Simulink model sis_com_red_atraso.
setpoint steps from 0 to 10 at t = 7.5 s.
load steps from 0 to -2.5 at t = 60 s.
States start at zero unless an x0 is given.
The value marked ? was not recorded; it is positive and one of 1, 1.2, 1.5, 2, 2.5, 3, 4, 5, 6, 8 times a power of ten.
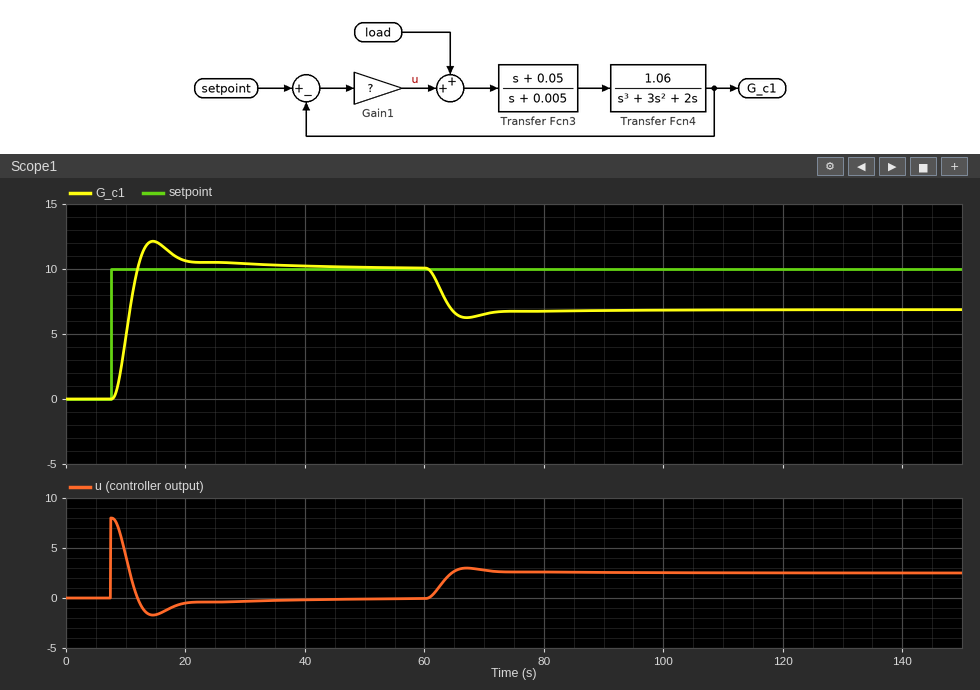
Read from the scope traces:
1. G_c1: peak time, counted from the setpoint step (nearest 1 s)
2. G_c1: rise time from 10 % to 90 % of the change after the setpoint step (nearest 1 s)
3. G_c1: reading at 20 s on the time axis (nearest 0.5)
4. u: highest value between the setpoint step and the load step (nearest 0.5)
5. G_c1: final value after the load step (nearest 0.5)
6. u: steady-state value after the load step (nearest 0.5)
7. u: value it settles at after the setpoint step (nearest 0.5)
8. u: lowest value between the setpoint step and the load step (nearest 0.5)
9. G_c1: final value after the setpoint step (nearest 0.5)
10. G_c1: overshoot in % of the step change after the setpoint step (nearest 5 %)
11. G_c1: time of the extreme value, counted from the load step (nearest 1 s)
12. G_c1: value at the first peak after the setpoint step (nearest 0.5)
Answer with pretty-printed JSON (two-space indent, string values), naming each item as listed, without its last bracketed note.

{
  "G_c1: peak time, counted from the setpoint step": "7 s",
  "G_c1: rise time from 10 % to 90 % of the change after the setpoint step": "3 s",
  "G_c1: reading at 20 s on the time axis": "10.5",
  "u: highest value between the setpoint step and the load step": "8.0",
  "G_c1: final value after the load step": "7.0",
  "u: steady-state value after the load step": "2.5",
  "u: value it settles at after the setpoint step": "0.0",
  "u: lowest value between the setpoint step and the load step": "-1.5",
  "G_c1: final value after the setpoint step": "10.0",
  "G_c1: overshoot in % of the step change after the setpoint step": "20 %",
  "G_c1: time of the extreme value, counted from the load step": "7 s",
  "G_c1: value at the first peak after the setpoint step": "12.0"
}
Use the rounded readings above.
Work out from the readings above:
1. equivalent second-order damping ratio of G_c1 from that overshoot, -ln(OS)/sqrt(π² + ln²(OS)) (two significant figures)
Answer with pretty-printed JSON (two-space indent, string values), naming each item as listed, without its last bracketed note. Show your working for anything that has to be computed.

{
  "equivalent second-order damping ratio of G_c1 from that overshoot, -ln(OS)/sqrt(π² + ln²(OS))": "ln(0.2) = -1.609; 1.609 / sqrt(9.870 + 2.590) = 0.46"
}
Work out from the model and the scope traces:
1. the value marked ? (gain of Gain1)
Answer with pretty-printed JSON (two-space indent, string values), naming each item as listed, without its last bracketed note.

{
  "the value marked ?": "0.8"
}
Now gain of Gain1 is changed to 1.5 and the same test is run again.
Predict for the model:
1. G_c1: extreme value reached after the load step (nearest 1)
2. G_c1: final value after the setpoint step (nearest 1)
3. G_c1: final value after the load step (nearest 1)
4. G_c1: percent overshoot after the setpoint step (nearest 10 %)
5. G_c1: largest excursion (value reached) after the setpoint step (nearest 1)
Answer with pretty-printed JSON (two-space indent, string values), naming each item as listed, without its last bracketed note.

{
  "G_c1: extreme value reached after the load step": "8",
  "G_c1: final value after the setpoint step": "10",
  "G_c1: final value after the load step": "8",
  "G_c1: percent overshoot after the setpoint step": "40 %",
  "G_c1: largest excursion (value reached) after the setpoint step": "14"
}
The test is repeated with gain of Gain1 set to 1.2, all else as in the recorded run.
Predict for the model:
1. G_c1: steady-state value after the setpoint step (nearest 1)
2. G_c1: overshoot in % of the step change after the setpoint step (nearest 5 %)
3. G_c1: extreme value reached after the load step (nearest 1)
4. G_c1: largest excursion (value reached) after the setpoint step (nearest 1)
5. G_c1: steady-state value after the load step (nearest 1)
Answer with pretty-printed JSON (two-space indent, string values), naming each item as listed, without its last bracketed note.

{
  "G_c1: steady-state value after the setpoint step": "10",
  "G_c1: overshoot in % of the step change after the setpoint step": "30 %",
  "G_c1: extreme value reached after the load step": "7",
  "G_c1: largest excursion (value reached) after the setpoint step": "13",
  "G_c1: steady-state value after the load step": "8"
}
